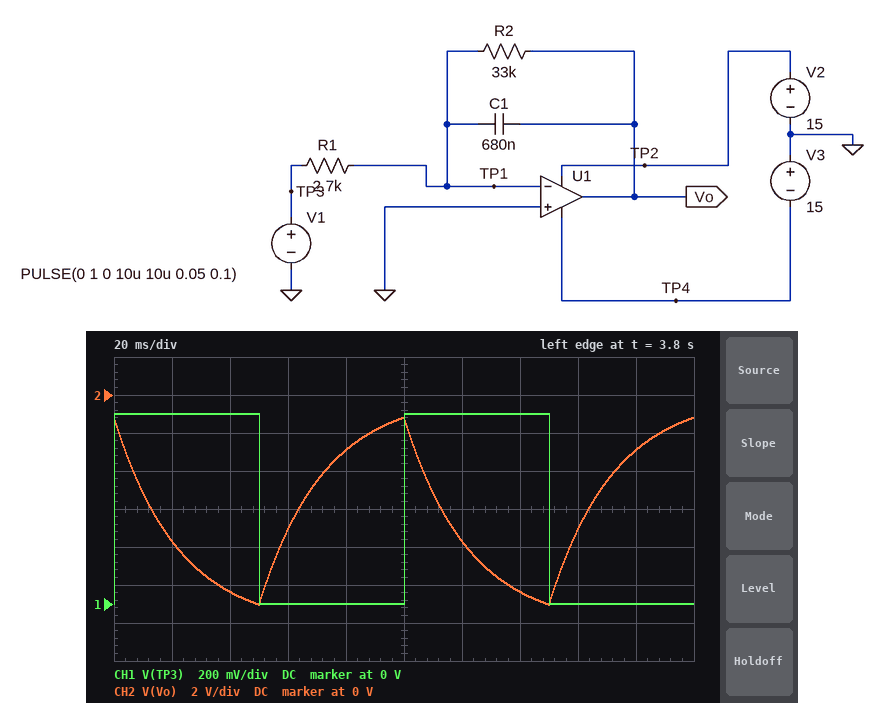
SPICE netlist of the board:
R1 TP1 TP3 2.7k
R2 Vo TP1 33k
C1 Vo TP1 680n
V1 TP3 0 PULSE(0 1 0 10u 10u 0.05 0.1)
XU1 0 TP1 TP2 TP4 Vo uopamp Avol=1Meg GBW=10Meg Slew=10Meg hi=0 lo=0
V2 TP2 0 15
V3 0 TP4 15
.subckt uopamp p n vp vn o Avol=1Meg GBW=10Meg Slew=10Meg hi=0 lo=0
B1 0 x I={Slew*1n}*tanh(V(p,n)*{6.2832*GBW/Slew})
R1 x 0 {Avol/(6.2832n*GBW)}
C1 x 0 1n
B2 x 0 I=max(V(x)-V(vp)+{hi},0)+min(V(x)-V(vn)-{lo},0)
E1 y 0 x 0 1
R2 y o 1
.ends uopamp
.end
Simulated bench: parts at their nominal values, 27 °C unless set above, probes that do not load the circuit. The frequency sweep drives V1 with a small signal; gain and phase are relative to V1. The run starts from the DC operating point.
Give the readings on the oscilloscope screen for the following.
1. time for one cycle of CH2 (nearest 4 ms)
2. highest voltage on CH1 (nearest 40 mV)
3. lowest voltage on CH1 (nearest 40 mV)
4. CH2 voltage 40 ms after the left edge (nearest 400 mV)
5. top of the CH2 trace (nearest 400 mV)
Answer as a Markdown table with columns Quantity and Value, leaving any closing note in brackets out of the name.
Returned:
| Quantity | Value |
|---|---|
| time for one cycle of CH2 | 100 ms |
| highest voltage on CH1 | 1.00 V |
| lowest voltage on CH1 | 0 V |
| CH2 voltage 40 ms after the left edge | -10.4 V |
| top of the CH2 trace | -1.2 V |
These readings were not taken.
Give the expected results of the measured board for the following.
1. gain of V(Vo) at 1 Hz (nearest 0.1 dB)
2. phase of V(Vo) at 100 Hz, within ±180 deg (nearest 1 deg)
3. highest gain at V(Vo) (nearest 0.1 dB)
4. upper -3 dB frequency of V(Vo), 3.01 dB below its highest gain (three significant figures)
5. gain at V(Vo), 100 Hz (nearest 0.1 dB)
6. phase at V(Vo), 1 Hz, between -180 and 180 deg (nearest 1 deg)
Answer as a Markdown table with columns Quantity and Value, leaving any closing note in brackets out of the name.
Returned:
| Quantity | Value |
|---|---|
| gain of V(Vo) at 1 Hz | 21.7 dB |
| phase of V(Vo) at 100 Hz, within ±180 deg | 94 deg |
| highest gain at V(Vo) | 21.7 dB |
| upper -3 dB frequency of V(Vo), 3.01 dB below its highest gain | 7.09 Hz |
| gain at V(Vo), 100 Hz | -1.3 dB |
| phase at V(Vo), 1 Hz, between -180 and 180 deg | 172 deg |
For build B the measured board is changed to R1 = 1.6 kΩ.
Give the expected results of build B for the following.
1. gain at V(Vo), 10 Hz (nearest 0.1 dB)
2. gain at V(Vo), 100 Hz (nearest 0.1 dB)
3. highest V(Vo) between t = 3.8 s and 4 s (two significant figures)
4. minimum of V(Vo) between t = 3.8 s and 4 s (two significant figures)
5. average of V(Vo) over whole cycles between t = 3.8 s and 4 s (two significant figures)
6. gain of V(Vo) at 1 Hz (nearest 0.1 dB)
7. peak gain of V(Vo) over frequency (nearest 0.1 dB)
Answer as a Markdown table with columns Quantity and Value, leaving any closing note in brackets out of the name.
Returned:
| Quantity | Value |
|---|---|
| gain at V(Vo), 10 Hz | 21.5 dB |
| gain at V(Vo), 100 Hz | 3.3 dB |
| highest V(Vo) between t = 3.8 s and 4 s | -1.6 V |
| minimum of V(Vo) between t = 3.8 s and 4 s | -15 V |
| average of V(Vo) over whole cycles between t = 3.8 s and 4 s | -9.1 V |
| gain of V(Vo) at 1 Hz | 26.2 dB |
| peak gain of V(Vo) over frequency | 26.3 dB |
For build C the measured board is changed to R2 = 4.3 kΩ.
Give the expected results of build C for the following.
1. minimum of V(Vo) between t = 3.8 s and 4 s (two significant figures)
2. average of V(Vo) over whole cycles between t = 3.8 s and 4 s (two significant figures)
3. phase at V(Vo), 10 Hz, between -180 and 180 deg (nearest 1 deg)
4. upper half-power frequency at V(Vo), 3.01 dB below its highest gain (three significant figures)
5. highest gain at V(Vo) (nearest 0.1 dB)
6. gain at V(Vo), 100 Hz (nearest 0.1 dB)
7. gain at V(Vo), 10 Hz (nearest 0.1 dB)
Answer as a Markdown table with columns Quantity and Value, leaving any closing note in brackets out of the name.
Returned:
| Quantity | Value |
|---|---|
| minimum of V(Vo) between t = 3.8 s and 4 s | -1.6 V |
| average of V(Vo) over whole cycles between t = 3.8 s and 4 s | -800 mV |
| phase at V(Vo), 10 Hz, between -180 and 180 deg | 170 deg |
| upper half-power frequency at V(Vo), 3.01 dB below its highest gain | 54.4 Hz |
| highest gain at V(Vo) | 4.0 dB |
| gain at V(Vo), 100 Hz | -2.4 dB |
| gain at V(Vo), 10 Hz | 3.9 dB |
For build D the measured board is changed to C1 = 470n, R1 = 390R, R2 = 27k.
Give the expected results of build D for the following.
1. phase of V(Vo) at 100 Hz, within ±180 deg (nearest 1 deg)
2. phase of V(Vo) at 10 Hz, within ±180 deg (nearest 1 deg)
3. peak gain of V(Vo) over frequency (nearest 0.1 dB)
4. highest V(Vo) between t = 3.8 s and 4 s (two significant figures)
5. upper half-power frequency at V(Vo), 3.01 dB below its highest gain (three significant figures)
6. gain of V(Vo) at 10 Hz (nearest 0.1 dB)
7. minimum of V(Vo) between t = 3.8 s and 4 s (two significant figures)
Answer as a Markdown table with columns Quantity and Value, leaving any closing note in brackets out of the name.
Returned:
| Quantity | Value |
|---|---|
| phase of V(Vo) at 100 Hz, within ±180 deg | 97 deg |
| phase of V(Vo) at 10 Hz, within ±180 deg | 141 deg |
| peak gain of V(Vo) over frequency | 36.8 dB |
| highest V(Vo) between t = 3.8 s and 4 s | -300 mV |
| upper half-power frequency at V(Vo), 3.01 dB below its highest gain | 12.5 Hz |
| gain of V(Vo) at 10 Hz | 34.7 dB |
| minimum of V(Vo) between t = 3.8 s and 4 s | -15 V |
